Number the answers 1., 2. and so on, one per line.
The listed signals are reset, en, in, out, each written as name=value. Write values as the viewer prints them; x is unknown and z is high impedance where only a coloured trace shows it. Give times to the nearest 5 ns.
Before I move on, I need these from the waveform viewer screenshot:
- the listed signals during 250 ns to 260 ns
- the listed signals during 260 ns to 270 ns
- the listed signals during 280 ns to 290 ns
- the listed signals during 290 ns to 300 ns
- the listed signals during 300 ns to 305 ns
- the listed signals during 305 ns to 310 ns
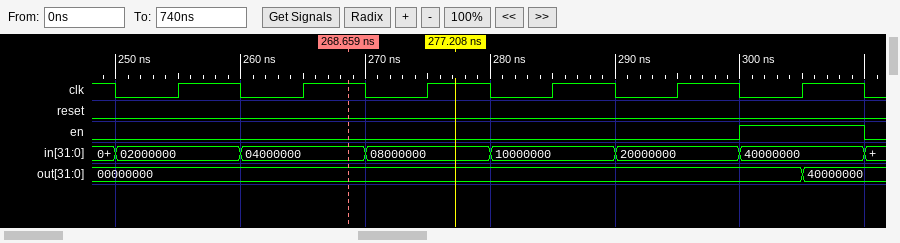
1. reset=0, en=0, in=02000000, out=00000000
2. reset=0, en=0, in=04000000, out=00000000
3. reset=0, en=0, in=10000000, out=00000000
4. reset=0, en=0, in=20000000, out=00000000
5. reset=0, en=1, in=40000000, out=00000000
6. reset=0, en=1, in=40000000, out=40000000
